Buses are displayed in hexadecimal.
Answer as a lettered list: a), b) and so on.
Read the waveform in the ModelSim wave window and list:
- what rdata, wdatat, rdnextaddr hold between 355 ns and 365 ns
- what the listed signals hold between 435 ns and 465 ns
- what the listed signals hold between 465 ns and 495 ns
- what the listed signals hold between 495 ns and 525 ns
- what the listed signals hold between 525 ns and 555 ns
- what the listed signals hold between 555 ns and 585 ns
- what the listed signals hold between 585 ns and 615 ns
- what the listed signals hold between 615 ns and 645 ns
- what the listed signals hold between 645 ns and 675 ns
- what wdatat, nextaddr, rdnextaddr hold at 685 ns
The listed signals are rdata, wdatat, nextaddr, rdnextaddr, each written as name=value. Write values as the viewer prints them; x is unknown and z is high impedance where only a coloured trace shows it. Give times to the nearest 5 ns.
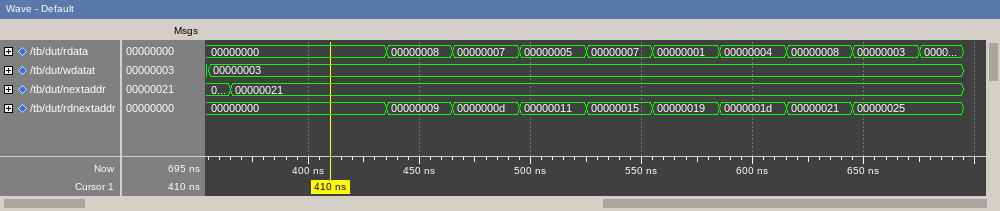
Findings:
a) rdata=00000000, wdatat=00000003, rdnextaddr=00000000
b) rdata=00000008, wdatat=00000003, nextaddr=00000021, rdnextaddr=00000009
c) rdata=00000007, wdatat=00000003, nextaddr=00000021, rdnextaddr=0000000d
d) rdata=00000005, wdatat=00000003, nextaddr=00000021, rdnextaddr=00000011
e) rdata=00000007, wdatat=00000003, nextaddr=00000021, rdnextaddr=00000015
f) rdata=00000001, wdatat=00000003, nextaddr=00000021, rdnextaddr=00000019
g) rdata=00000004, wdatat=00000003, nextaddr=00000021, rdnextaddr=0000001d
h) rdata=00000008, wdatat=00000003, nextaddr=00000021, rdnextaddr=00000021
i) rdata=00000003, wdatat=00000003, nextaddr=00000021, rdnextaddr=00000025
j) wdatat=00000003, nextaddr=00000021, rdnextaddr=00000025
